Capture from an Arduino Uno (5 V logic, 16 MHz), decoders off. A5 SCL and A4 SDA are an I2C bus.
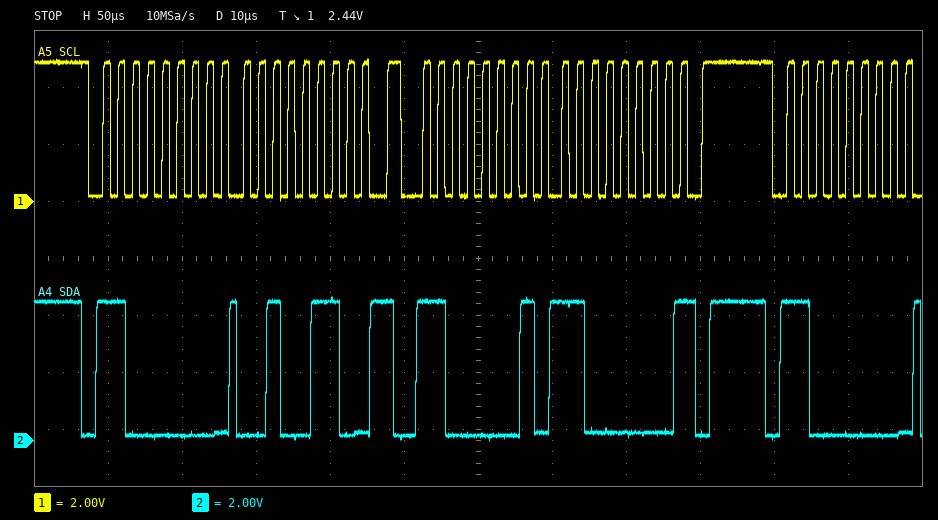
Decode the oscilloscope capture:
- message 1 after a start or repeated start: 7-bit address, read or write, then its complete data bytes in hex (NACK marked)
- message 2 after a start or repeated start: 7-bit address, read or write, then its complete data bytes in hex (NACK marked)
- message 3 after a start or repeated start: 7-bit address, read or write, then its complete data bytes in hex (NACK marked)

0x60 write: 26
0x60 read: C0 NACK
0x60 write
